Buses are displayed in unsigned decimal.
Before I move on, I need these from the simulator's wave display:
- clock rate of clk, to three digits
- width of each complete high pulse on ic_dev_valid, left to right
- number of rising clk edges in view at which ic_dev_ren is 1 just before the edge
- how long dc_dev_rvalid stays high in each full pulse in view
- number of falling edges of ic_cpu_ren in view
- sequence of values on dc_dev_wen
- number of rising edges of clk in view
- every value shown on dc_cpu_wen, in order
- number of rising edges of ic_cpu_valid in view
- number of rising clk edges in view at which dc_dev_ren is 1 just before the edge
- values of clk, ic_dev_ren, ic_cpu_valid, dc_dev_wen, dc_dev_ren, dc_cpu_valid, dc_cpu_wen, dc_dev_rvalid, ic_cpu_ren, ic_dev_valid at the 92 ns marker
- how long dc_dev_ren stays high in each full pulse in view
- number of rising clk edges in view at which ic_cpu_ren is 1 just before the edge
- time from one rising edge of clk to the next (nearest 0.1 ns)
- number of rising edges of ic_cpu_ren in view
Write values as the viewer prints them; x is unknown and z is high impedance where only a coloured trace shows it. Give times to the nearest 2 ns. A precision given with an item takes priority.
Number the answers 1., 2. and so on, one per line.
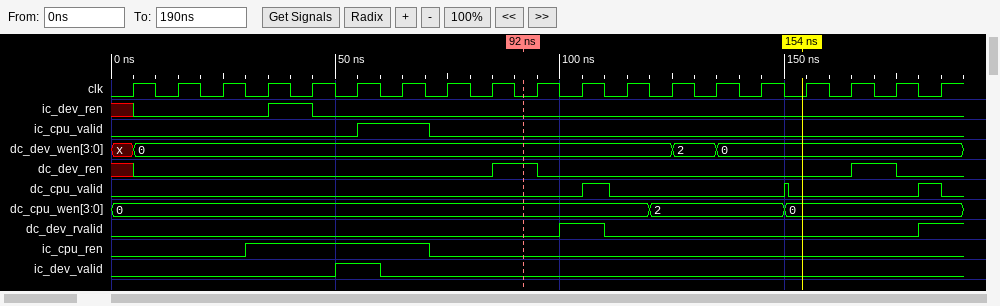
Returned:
1. 100 MHz
2. 10 ns
3. 1
4. 10 ns
5. 1
6. x, 0, 2, 0
7. 19
8. 0, 2, 0
9. 1
10. 2
11. clk=0, ic_dev_ren=0, ic_cpu_valid=0, dc_dev_wen=0, dc_dev_ren=1, dc_cpu_valid=0, dc_cpu_wen=0, dc_dev_rvalid=0, ic_cpu_ren=0, ic_dev_valid=0
12. 10 ns, 10 ns
13. 4
14. 10 ns
15. 1
